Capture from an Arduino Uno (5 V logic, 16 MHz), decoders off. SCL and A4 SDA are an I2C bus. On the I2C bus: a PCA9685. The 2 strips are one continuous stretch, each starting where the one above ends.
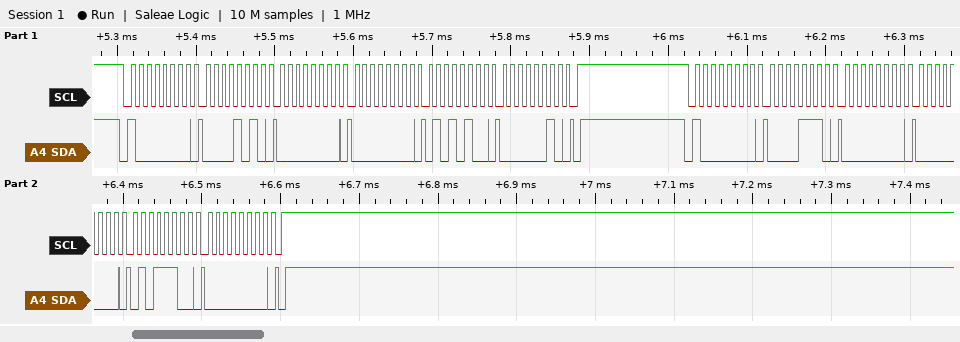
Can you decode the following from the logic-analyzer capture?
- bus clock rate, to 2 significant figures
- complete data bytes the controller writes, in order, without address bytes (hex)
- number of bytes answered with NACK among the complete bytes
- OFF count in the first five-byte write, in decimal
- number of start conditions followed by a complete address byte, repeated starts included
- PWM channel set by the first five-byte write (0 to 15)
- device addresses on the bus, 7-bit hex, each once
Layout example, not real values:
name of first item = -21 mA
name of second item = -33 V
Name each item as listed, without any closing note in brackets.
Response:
bus clock rate, to 2 significant figures = 100 kHz
complete data bytes the controller writes, in order, without address bytes = 0A 00 00 54 02 0E 00 00 5C 00
number of bytes answered with NACK among the complete bytes = 0
OFF count in the first five-byte write, in decimal = 596
number of start conditions followed by a complete address byte, repeated starts included = 2
PWM channel set by the first five-byte write = 1
device addresses on the bus, 7-bit hex, each once = 0x40
